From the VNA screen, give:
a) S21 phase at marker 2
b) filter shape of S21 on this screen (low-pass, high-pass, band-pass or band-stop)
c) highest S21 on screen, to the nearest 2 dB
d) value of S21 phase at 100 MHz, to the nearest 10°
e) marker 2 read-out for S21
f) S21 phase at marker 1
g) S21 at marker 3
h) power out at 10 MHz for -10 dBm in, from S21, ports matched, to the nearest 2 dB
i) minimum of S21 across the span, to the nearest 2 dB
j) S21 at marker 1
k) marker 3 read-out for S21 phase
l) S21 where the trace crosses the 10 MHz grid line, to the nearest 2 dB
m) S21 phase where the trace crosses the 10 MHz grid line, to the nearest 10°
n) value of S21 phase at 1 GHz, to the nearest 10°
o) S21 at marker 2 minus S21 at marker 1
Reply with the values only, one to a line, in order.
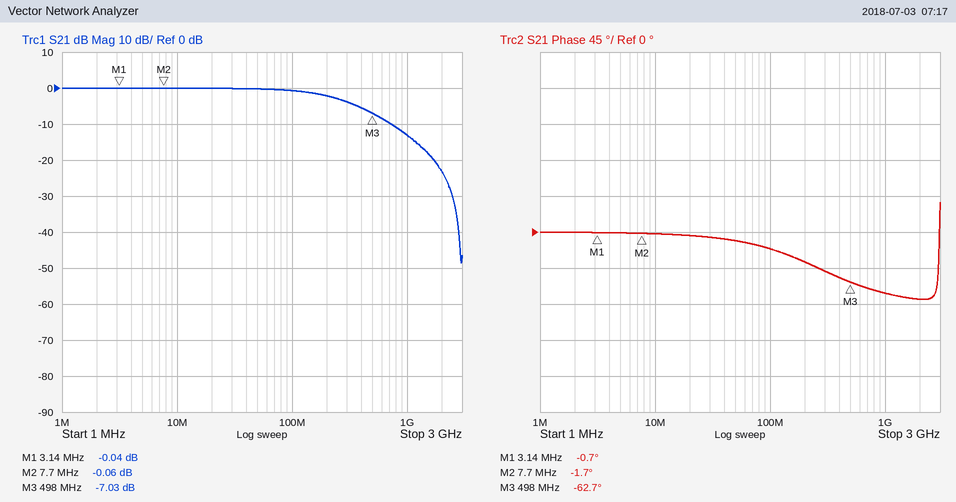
-1.7°
low-pass
0 dB
-20°
-0.06 dB
-0.7°
-7.03 dB
-10 dBm
-48 dB
-0.04 dB
-62.7°
0 dB
0°
-80°
-0.02 dB
